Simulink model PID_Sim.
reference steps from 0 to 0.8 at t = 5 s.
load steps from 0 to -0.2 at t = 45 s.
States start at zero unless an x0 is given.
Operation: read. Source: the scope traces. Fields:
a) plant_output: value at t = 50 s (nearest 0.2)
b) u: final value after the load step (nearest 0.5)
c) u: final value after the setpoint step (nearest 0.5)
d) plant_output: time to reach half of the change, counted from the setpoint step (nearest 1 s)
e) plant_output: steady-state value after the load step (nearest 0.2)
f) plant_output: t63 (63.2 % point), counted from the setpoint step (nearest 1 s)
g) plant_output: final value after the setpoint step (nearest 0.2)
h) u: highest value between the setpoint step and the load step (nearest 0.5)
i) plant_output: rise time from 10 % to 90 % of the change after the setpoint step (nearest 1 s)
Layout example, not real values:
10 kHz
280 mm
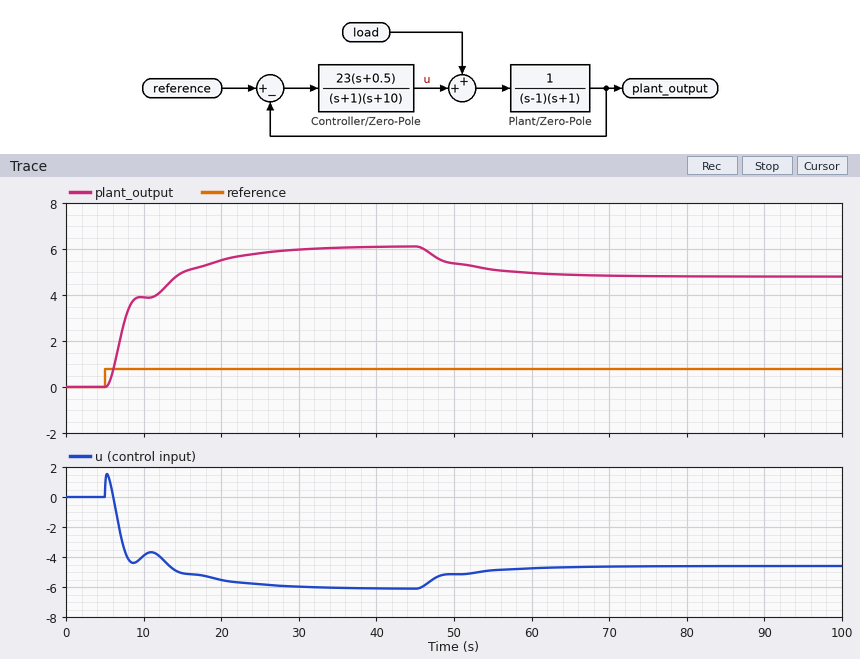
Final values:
5.4
-4.5
-6.0
3 s
4.8
4 s
6.2
1.5
14 s
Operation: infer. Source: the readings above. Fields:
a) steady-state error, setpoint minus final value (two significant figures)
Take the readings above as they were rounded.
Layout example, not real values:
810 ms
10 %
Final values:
-5.4
